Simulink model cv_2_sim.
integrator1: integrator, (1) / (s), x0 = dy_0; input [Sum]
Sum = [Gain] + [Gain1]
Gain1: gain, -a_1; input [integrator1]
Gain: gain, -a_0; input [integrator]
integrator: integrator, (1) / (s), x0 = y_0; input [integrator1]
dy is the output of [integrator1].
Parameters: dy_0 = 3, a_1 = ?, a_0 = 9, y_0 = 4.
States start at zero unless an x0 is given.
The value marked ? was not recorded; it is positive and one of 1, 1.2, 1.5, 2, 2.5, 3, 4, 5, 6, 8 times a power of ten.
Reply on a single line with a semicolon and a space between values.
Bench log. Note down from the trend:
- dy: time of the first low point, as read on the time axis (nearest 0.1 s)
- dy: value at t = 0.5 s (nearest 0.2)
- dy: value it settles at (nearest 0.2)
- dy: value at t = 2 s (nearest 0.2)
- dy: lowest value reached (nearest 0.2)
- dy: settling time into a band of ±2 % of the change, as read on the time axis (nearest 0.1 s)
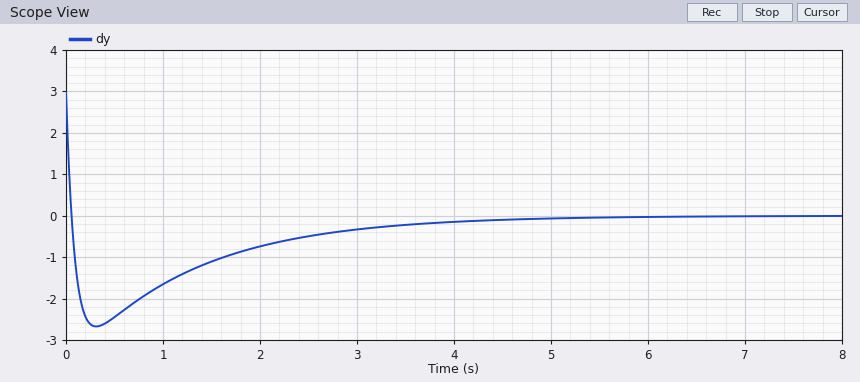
0.3 s; -2.4; 0.0; -0.8; -2.6; 5.1 s
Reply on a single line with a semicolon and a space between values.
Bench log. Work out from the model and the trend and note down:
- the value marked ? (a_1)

12
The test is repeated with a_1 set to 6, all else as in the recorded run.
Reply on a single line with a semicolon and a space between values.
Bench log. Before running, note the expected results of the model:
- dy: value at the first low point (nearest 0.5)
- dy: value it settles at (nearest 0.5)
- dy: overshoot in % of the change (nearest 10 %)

-4.5; 0.0; 150 %
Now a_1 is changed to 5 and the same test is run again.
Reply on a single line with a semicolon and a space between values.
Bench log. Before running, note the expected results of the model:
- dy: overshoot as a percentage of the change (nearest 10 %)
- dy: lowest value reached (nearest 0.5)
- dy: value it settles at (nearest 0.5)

170 %; -5.0; 0.0
